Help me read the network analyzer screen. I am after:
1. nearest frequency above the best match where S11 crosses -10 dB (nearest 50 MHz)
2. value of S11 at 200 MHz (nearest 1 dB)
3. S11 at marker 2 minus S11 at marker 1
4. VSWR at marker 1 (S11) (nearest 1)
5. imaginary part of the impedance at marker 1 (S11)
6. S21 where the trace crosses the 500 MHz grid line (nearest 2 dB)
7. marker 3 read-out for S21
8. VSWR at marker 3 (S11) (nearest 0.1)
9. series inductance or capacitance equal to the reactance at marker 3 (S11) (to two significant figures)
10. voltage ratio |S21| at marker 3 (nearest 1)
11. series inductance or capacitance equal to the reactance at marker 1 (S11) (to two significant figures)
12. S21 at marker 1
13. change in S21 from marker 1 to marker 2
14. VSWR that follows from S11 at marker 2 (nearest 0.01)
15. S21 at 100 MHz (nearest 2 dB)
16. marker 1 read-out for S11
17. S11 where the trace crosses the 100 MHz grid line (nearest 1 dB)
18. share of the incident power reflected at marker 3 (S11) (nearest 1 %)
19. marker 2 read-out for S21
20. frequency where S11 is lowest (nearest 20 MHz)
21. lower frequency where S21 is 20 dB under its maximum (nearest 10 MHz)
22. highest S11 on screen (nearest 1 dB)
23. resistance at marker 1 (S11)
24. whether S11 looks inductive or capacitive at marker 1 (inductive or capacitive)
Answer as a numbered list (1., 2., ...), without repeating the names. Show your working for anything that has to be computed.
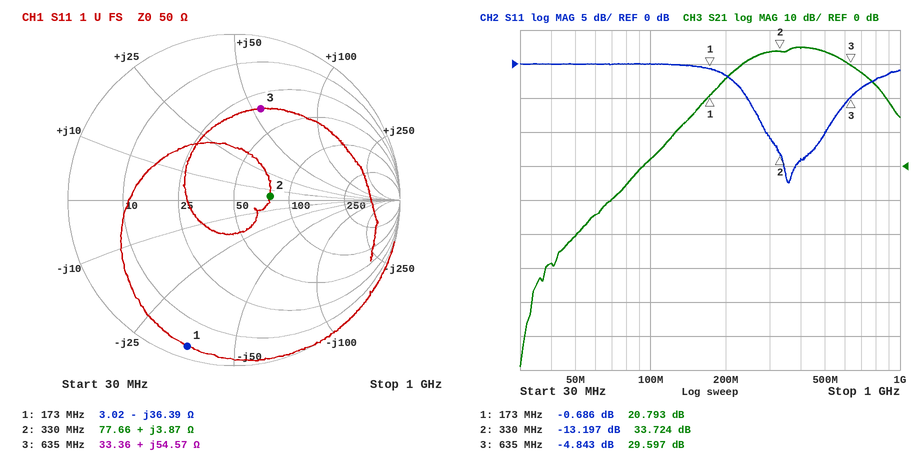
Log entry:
1. 500 MHz
2. -2 dB
3. -13.197 − (-0.686) = -12.511 dB
4. (1 + 0.9241)/(1 − 0.9241) ≈ 25
5. -36.39 Ω
6. 34 dB
7. 29.597 dB
8. 3.7
9. L = 54.57 Ω/(2π × 635 MHz) ≈ 14 nH
10. 10^(29.597/20) ≈ 30
11. C = 1/(2π × 173 MHz × 36.39 Ω) ≈ 25 pF
12. 20.793 dB
13. 33.724 − (20.793) = 12.931 dB
14. (1 + 0.2189)/(1 − 0.2189) ≈ 1.56
15. 2 dB
16. -0.686 dB
17. 0 dB
18. 10^(-4.843/10) ≈ 33 %
19. 33.724 dB
20. 360 MHz
21. 150 MHz
22. 0 dB
23. 3.02 Ω
24. capacitive
